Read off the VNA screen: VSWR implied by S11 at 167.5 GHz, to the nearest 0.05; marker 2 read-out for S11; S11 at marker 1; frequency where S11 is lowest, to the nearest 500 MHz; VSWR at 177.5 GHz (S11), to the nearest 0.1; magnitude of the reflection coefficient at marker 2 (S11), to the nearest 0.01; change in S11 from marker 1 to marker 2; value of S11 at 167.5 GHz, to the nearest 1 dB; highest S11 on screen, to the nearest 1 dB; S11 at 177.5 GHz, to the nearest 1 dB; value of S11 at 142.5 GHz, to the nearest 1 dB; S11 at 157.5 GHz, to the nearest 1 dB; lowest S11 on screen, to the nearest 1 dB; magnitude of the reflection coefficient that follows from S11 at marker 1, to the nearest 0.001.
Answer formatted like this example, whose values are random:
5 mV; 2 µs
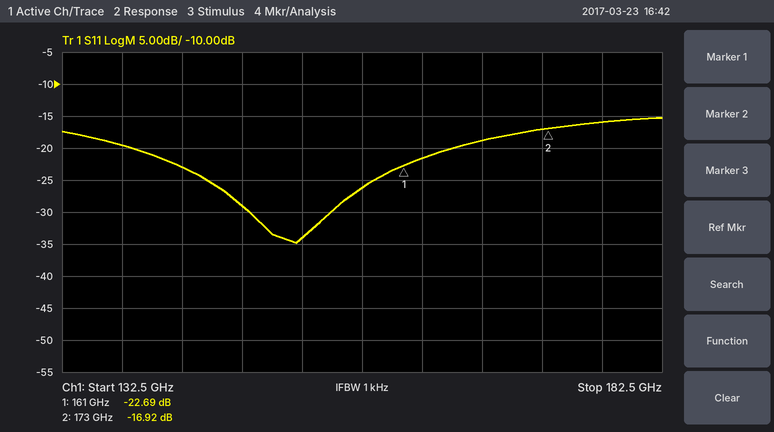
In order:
1.25; -16.92 dB; -22.69 dB; 152.0 GHz; 1.4; 0.14; 5.77 dB; -19 dB; -15 dB; -16 dB; -23 dB; -26 dB; -35 dB; 0.073
